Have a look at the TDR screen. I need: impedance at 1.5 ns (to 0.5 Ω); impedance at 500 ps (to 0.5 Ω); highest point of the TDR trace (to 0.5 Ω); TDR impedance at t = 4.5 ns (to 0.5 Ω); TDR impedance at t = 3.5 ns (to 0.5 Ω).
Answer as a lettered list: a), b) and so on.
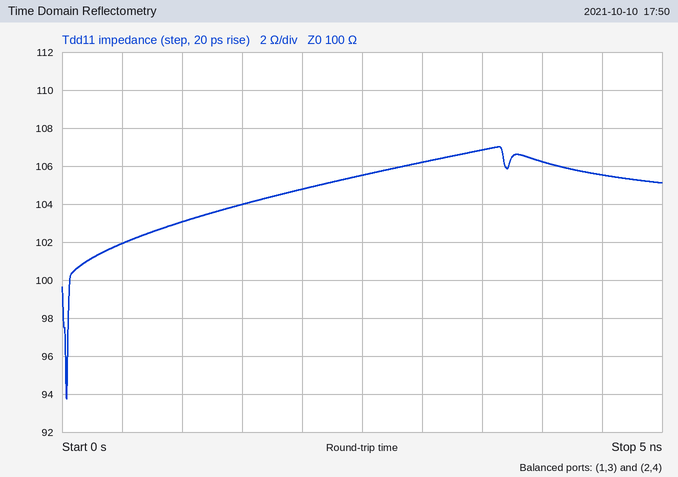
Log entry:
a) 104.0 Ω
b) 102.0 Ω
c) 107.0 Ω
d) 105.5 Ω
e) 107.0 Ω
